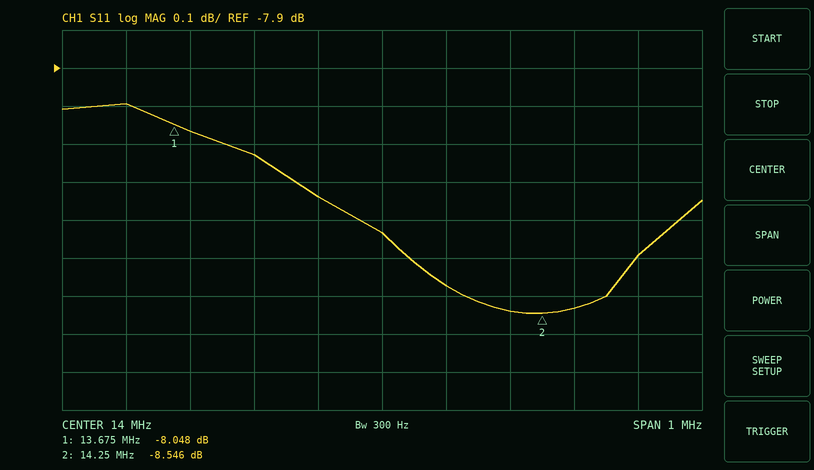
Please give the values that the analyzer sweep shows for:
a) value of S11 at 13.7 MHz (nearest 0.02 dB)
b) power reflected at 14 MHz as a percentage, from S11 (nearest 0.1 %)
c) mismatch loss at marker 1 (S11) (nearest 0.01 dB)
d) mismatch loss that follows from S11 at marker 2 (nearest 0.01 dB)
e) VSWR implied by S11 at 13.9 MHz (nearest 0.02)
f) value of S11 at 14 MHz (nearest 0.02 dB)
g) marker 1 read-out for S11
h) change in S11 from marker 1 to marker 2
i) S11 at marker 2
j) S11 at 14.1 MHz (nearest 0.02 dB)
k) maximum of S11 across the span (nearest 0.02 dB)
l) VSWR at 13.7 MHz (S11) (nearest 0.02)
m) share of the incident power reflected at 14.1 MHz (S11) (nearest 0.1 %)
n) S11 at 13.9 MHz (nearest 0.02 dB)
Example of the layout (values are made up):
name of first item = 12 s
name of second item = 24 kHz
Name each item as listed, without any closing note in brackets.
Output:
value of S11 at 13.7 MHz = -8.06 dB
power reflected at 14 MHz as a percentage, from S11 = 14.7 %
mismatch loss at marker 1 (S11) = 0.74 dB
mismatch loss that follows from S11 at marker 2 = 0.65 dB
VSWR implied by S11 at 13.9 MHz = 2.26
value of S11 at 14 MHz = -8.34 dB
marker 1 read-out for S11 = -8.048 dB
change in S11 from marker 1 to marker 2 = -0.498 dB
S11 at marker 2 = -8.546 dB
S11 at 14.1 MHz = -8.48 dB
maximum of S11 across the span = -8.00 dB
VSWR at 13.7 MHz (S11) = 2.30
share of the incident power reflected at 14.1 MHz (S11) = 14.2 %
S11 at 13.9 MHz = -8.24 dB
